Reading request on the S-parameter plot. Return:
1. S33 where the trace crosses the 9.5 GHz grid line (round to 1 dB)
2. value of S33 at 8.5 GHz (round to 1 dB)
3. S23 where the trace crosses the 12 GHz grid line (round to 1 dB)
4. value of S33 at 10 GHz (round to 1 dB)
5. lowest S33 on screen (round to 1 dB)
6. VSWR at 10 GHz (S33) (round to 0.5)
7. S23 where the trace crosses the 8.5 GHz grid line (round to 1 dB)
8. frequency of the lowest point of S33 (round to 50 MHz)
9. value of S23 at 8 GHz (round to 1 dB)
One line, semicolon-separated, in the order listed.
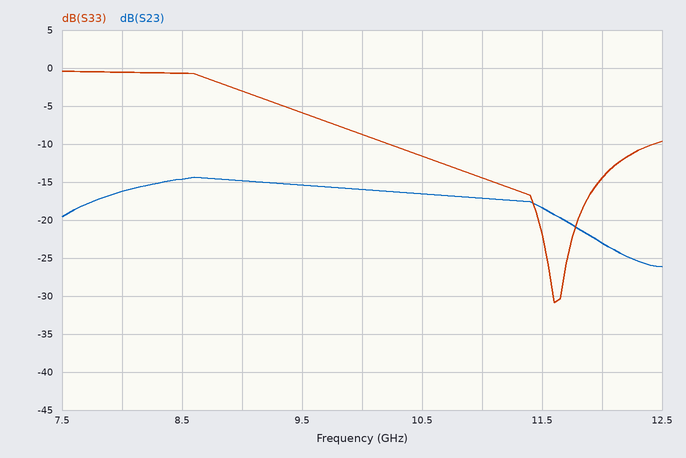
-6 dB; -1 dB; -23 dB; -9 dB; -31 dB; 2.0; -15 dB; 11.60 GHz; -16 dB
